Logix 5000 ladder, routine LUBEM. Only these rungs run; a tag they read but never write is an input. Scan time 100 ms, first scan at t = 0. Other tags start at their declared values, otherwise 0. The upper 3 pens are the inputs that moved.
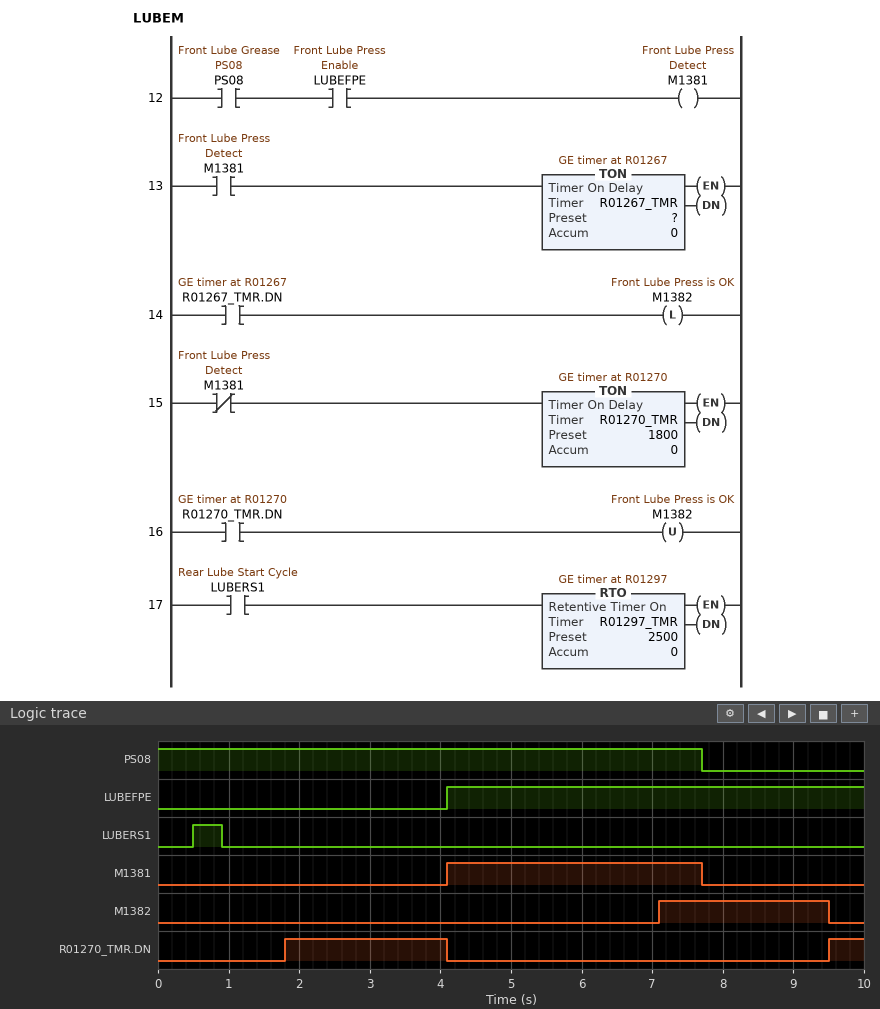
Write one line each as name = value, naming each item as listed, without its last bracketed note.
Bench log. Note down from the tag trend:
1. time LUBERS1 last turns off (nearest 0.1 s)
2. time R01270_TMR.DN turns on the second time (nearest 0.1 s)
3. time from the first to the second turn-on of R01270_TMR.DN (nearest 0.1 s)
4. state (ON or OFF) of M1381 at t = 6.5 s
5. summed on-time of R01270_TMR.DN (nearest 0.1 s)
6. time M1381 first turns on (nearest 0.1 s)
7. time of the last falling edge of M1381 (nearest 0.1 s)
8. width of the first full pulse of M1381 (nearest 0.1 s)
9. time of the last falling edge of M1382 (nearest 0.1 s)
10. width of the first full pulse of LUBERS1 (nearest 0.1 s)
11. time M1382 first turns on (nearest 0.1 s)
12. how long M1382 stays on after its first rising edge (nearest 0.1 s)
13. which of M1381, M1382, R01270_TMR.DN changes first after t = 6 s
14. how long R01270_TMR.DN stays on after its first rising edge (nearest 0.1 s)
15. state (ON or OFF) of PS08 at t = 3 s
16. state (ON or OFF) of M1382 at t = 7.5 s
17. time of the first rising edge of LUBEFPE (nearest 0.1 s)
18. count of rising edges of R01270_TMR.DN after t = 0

time LUBERS1 last turns off = 0.9 s
time R01270_TMR.DN turns on the second time = 9.5 s
time from the first to the second turn-on of R01270_TMR.DN = 7.7 s
state (ON or OFF) of M1381 at t = 6.5 s = ON
summed on-time of R01270_TMR.DN = 2.8 s
time M1381 first turns on = 4.1 s
time of the last falling edge of M1381 = 7.7 s
width of the first full pulse of M1381 = 3.6 s
time of the last falling edge of M1382 = 9.5 s
width of the first full pulse of LUBERS1 = 0.4 s
time M1382 first turns on = 7.1 s
how long M1382 stays on after its first rising edge = 2.4 s
which of M1381, M1382, R01270_TMR.DN changes first after t = 6 s = M1382
how long R01270_TMR.DN stays on after its first rising edge = 2.3 s
state (ON or OFF) of PS08 at t = 3 s = ON
state (ON or OFF) of M1382 at t = 7.5 s = ON
time of the first rising edge of LUBEFPE = 4.1 s
count of rising edges of R01270_TMR.DN after t = 0 = 2
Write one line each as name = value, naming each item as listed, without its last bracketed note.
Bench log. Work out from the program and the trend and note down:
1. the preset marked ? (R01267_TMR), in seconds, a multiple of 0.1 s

the preset marked ? (R01267_TMR), in seconds, a multiple of 0.1 s = 3.0 s
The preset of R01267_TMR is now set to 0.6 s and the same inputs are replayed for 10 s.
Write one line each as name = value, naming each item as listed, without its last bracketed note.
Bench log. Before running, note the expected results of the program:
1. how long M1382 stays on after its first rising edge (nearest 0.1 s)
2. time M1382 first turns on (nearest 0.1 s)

how long M1382 stays on after its first rising edge = 4.8 s
time M1382 first turns on = 4.7 s
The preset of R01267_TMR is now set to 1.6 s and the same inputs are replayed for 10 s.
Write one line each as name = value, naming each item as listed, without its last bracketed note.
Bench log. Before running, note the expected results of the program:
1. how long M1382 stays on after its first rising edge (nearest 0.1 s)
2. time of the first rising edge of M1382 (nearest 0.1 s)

how long M1382 stays on after its first rising edge = 3.8 s
time of the first rising edge of M1382 = 5.7 s
